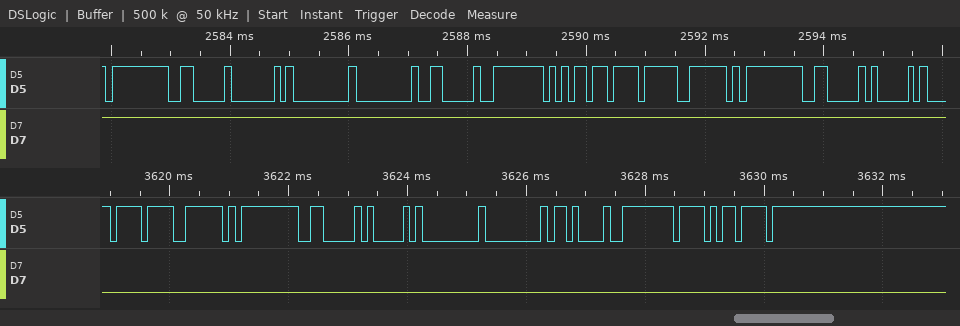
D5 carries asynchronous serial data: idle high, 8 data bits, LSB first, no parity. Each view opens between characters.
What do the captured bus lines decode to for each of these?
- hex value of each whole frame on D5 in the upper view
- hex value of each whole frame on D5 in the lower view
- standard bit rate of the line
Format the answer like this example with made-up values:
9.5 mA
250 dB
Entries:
FF, 06, 40, 00, 00, 06, FE, B5, EF, 7E, FF, 06, 41
EF, 7E, FF, 06, 41, 00, 00, 0B, FE, AF, EF
9600 baud
